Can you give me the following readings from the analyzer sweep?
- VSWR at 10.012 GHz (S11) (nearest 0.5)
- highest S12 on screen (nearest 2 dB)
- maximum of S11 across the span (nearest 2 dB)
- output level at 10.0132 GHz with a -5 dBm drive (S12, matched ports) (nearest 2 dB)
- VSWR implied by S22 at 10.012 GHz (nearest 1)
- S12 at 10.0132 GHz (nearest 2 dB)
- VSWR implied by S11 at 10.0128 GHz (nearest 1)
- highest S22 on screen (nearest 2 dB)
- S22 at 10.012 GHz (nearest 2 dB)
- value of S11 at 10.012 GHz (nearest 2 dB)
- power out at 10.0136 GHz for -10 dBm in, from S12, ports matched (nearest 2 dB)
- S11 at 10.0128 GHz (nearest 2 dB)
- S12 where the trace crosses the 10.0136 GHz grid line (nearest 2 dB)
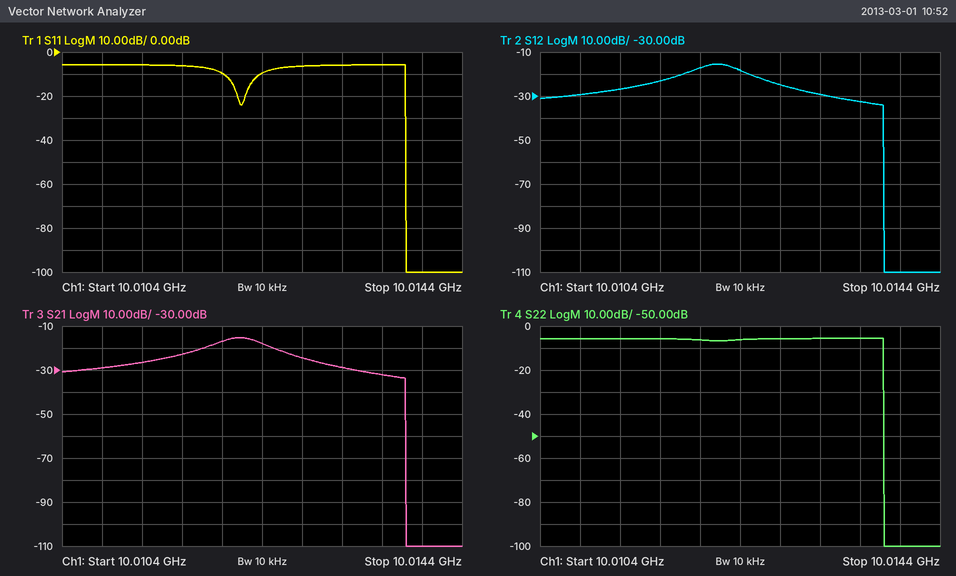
2.0
-16 dB
-6 dB
-34 dBm
3
-30 dB
3
-6 dB
-6 dB
-10 dB
-42 dBm
-6 dB
-32 dB
